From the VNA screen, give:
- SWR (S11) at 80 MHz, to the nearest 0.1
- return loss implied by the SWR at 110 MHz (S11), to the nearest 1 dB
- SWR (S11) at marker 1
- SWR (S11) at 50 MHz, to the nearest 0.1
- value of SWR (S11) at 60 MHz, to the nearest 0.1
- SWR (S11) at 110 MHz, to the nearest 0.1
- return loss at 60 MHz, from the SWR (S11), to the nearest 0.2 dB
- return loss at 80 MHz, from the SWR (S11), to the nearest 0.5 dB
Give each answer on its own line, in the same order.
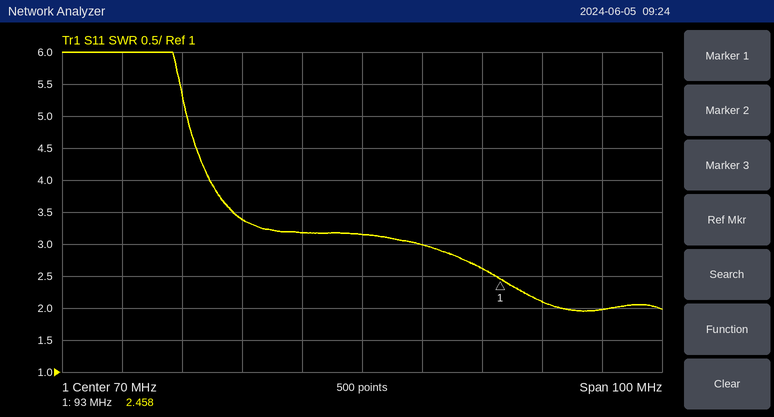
3.0
10 dB
2.458
3.4
3.2
2.0
5.6 dB
6.0 dB
